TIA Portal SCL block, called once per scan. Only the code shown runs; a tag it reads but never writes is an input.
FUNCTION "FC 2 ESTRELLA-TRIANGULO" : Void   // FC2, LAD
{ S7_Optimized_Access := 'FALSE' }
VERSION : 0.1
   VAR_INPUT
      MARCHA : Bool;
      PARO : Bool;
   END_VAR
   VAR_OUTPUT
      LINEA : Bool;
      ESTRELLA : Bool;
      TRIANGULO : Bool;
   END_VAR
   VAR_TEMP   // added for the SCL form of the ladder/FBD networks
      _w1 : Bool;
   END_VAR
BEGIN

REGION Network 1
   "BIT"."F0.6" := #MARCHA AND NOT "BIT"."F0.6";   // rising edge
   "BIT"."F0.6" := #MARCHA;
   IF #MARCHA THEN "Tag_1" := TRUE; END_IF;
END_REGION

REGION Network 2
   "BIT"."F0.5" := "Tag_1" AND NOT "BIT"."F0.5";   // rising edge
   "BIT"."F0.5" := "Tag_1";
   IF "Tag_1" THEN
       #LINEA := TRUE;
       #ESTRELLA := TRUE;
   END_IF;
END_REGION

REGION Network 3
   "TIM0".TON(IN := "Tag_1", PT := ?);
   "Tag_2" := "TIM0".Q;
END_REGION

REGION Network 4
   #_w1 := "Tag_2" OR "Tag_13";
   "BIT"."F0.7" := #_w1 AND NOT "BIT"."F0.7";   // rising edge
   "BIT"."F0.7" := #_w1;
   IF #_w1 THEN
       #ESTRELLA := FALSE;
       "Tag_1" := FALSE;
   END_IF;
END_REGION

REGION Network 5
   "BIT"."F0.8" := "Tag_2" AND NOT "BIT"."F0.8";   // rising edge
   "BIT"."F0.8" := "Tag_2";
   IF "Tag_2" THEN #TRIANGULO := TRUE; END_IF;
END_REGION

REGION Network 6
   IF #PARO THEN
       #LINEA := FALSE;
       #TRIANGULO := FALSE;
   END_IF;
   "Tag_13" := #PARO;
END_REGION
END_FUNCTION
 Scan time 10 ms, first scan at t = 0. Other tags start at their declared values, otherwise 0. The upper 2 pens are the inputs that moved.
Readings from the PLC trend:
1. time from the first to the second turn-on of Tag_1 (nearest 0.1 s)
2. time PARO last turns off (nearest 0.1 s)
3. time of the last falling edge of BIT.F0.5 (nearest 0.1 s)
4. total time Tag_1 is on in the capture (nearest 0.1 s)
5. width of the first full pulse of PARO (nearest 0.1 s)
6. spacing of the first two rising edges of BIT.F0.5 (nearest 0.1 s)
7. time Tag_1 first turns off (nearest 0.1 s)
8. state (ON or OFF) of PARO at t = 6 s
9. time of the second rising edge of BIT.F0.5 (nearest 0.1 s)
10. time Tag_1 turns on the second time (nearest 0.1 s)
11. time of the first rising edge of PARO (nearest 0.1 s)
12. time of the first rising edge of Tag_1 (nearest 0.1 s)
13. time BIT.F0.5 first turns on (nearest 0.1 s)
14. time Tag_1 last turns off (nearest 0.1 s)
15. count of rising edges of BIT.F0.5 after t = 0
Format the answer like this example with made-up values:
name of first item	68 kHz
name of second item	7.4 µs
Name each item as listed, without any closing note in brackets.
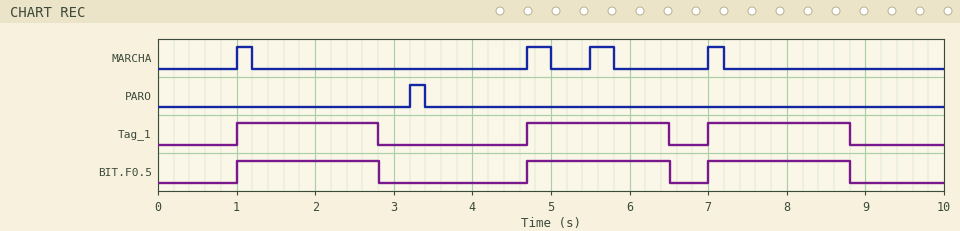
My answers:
time from the first to the second turn-on of Tag_1	3.7 s
time PARO last turns off	3.4 s
time of the last falling edge of BIT.F0.5	8.8 s
total time Tag_1 is on in the capture	5.4 s
width of the first full pulse of PARO	0.2 s
spacing of the first two rising edges of BIT.F0.5	3.7 s
time Tag_1 first turns off	2.8 s
state (ON or OFF) of PARO at t = 6 s	OFF
time of the second rising edge of BIT.F0.5	4.7 s
time Tag_1 turns on the second time	4.7 s
time of the first rising edge of PARO	3.2 s
time of the first rising edge of Tag_1	1.0 s
time BIT.F0.5 first turns on	1.0 s
time Tag_1 last turns off	8.8 s
count of rising edges of BIT.F0.5 after t = 0	3
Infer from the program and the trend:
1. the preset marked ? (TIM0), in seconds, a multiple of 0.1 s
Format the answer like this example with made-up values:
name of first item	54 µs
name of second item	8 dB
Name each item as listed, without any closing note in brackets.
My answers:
the preset marked ? (TIM0), in seconds, a multiple of 0.1 s	1.8 s
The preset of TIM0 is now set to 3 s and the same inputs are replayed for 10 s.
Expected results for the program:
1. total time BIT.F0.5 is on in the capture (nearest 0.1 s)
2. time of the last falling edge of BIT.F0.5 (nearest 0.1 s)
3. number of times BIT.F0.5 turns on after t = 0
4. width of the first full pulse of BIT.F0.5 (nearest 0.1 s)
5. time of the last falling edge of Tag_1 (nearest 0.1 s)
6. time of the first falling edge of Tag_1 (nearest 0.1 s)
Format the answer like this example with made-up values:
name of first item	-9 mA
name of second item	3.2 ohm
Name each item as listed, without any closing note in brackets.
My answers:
total time BIT.F0.5 is on in the capture	5.2 s
time of the last falling edge of BIT.F0.5	7.7 s
number of times BIT.F0.5 turns on after t = 0	2
width of the first full pulse of BIT.F0.5	2.2 s
time of the last falling edge of Tag_1	7.7 s
time of the first falling edge of Tag_1	3.2 s
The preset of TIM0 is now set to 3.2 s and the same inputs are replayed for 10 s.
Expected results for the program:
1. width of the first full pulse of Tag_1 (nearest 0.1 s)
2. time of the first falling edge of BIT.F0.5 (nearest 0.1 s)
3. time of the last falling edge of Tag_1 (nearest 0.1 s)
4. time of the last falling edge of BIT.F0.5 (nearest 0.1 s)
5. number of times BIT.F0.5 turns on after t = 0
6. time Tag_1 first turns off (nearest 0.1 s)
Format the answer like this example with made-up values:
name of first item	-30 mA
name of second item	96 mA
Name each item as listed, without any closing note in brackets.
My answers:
width of the first full pulse of Tag_1	2.2 s
time of the first falling edge of BIT.F0.5	3.2 s
time of the last falling edge of Tag_1	7.9 s
time of the last falling edge of BIT.F0.5	7.9 s
number of times BIT.F0.5 turns on after t = 0	2
time Tag_1 first turns off	3.2 s
